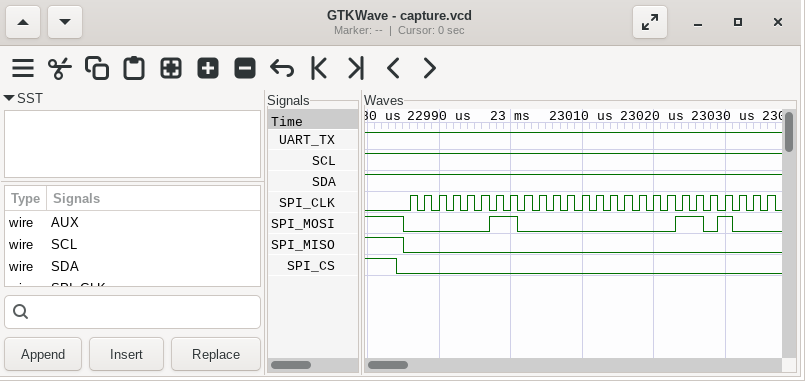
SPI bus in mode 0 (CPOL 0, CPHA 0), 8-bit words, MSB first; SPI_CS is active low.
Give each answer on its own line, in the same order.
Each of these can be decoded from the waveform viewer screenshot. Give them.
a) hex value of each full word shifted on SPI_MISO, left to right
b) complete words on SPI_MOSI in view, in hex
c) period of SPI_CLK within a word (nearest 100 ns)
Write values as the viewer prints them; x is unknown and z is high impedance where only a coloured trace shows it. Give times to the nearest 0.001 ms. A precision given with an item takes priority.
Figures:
00, 00, 00
03, 00, 1A
2000 ns
